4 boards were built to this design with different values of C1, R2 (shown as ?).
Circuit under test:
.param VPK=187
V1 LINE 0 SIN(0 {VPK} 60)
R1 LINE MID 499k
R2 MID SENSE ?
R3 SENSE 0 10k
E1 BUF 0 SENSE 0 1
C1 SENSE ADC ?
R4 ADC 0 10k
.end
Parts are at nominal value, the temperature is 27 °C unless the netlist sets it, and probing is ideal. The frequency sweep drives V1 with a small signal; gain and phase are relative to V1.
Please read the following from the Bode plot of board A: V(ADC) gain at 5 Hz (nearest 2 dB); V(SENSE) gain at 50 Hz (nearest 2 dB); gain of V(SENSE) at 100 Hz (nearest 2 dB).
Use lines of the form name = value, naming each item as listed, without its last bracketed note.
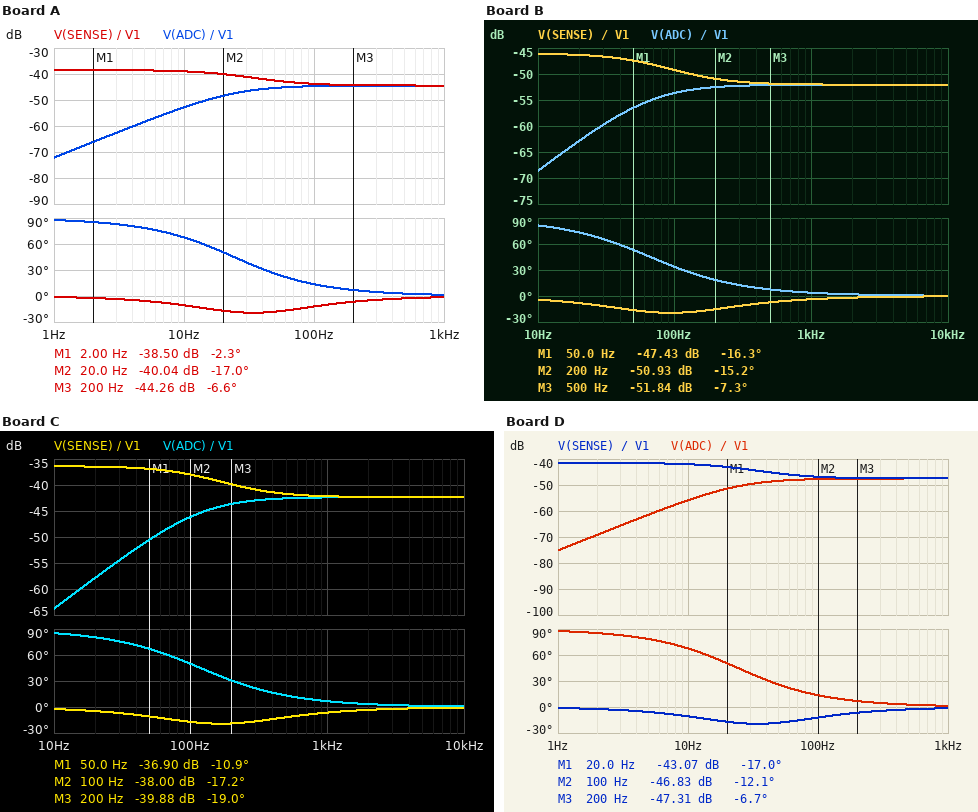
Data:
V(ADC) gain at 5 Hz = -58 dB
V(SENSE) gain at 50 Hz = -42 dB
gain of V(SENSE) at 100 Hz = -44 dB
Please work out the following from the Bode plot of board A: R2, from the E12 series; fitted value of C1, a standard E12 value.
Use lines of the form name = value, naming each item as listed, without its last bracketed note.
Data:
R2, from the E12 series = 330 kΩ
fitted value of C1, a standard E12 value = 330 nF
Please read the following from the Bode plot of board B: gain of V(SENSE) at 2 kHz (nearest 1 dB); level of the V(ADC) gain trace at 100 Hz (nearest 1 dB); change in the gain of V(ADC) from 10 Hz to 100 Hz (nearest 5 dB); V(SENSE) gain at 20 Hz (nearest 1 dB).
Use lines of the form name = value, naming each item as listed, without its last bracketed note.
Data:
gain of V(SENSE) at 2 kHz = -52 dB
level of the V(ADC) gain trace at 100 Hz = -54 dB
change in the gain of V(ADC) from 10 Hz to 100 Hz = 15 dB
V(SENSE) gain at 20 Hz = -46 dB
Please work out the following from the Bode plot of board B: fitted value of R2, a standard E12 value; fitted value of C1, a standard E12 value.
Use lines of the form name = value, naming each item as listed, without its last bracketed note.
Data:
fitted value of R2, a standard E12 value = 1.5 MΩ
fitted value of C1, a standard E12 value = 120 nF
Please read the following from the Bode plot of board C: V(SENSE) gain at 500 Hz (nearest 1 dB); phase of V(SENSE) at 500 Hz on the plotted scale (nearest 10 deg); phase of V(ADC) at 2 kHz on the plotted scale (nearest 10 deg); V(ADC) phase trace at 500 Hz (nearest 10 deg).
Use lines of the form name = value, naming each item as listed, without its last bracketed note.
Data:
V(SENSE) gain at 500 Hz = -42 dB
phase of V(SENSE) at 500 Hz on the plotted scale = -10 deg
phase of V(ADC) at 2 kHz on the plotted scale = 0 deg
V(ADC) phase trace at 500 Hz = 10 deg
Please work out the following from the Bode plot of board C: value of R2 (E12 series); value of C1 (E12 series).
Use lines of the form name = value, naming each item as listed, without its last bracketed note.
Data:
value of R2 = 150 kΩ
value of C1 = 68 nF
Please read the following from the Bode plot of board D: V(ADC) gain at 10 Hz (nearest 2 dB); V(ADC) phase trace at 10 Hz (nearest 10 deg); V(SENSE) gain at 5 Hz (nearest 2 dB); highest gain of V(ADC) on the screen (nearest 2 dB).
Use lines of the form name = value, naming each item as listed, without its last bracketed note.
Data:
V(ADC) gain at 10 Hz = -56 dB
V(ADC) phase trace at 10 Hz = 70 deg
V(SENSE) gain at 5 Hz = -42 dB
highest gain of V(ADC) on the screen = -48 dB
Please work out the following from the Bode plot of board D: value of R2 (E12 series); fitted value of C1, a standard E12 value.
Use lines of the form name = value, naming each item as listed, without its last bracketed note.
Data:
value of R2 = 680 kΩ
fitted value of C1, a standard E12 value = 330 nF
